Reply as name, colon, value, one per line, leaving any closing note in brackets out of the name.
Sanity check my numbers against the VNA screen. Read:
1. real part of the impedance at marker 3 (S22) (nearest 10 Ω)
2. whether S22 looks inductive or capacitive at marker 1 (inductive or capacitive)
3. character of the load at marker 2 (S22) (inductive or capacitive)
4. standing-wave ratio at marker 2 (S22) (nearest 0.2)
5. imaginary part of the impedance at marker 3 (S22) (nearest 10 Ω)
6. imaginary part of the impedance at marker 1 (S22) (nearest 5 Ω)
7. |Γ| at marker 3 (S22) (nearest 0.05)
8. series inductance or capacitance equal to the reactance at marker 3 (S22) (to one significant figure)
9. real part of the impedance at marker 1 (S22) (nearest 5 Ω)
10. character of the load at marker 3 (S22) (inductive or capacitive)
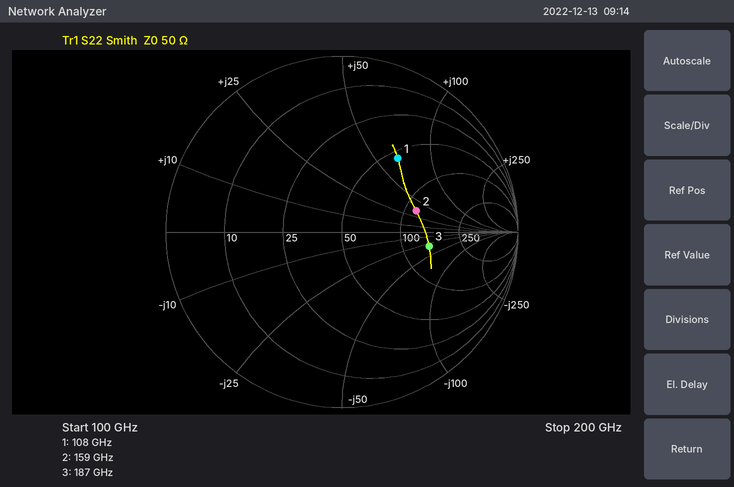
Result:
real part of the impedance at marker 3 (S22): 140 Ω
whether S22 looks inductive or capacitive at marker 1: inductive
character of the load at marker 2 (S22): inductive
standing-wave ratio at marker 2 (S22): 2.6
imaginary part of the impedance at marker 3 (S22): -30 Ω
imaginary part of the impedance at marker 1 (S22): +65 Ω
|Γ| at marker 3 (S22): 0.50
series inductance or capacitance equal to the reactance at marker 3 (S22): 30 fF
real part of the impedance at marker 1 (S22): 55 Ω
character of the load at marker 3 (S22): capacitive
